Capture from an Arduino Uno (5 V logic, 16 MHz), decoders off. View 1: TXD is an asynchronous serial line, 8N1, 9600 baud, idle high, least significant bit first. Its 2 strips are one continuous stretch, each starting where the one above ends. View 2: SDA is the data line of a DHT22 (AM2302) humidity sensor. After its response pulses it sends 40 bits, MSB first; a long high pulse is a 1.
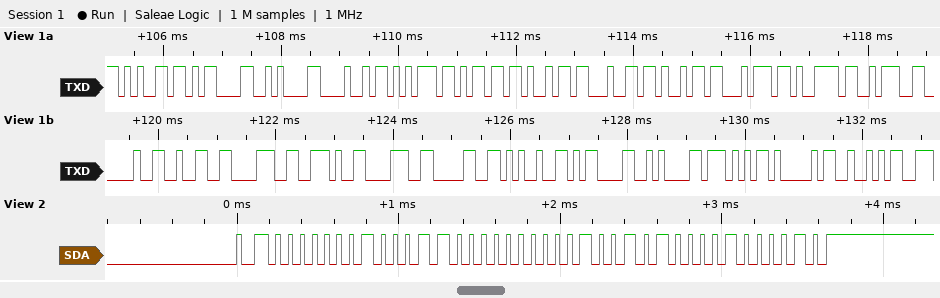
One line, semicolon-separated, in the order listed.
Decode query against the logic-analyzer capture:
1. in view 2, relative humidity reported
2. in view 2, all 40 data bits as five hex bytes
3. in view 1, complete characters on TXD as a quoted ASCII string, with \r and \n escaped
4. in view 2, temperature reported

28.0 %; 01 18 01 28 42; "e\r\nHumidity: 28.80%\r\nWAR"; 29.6 °C
